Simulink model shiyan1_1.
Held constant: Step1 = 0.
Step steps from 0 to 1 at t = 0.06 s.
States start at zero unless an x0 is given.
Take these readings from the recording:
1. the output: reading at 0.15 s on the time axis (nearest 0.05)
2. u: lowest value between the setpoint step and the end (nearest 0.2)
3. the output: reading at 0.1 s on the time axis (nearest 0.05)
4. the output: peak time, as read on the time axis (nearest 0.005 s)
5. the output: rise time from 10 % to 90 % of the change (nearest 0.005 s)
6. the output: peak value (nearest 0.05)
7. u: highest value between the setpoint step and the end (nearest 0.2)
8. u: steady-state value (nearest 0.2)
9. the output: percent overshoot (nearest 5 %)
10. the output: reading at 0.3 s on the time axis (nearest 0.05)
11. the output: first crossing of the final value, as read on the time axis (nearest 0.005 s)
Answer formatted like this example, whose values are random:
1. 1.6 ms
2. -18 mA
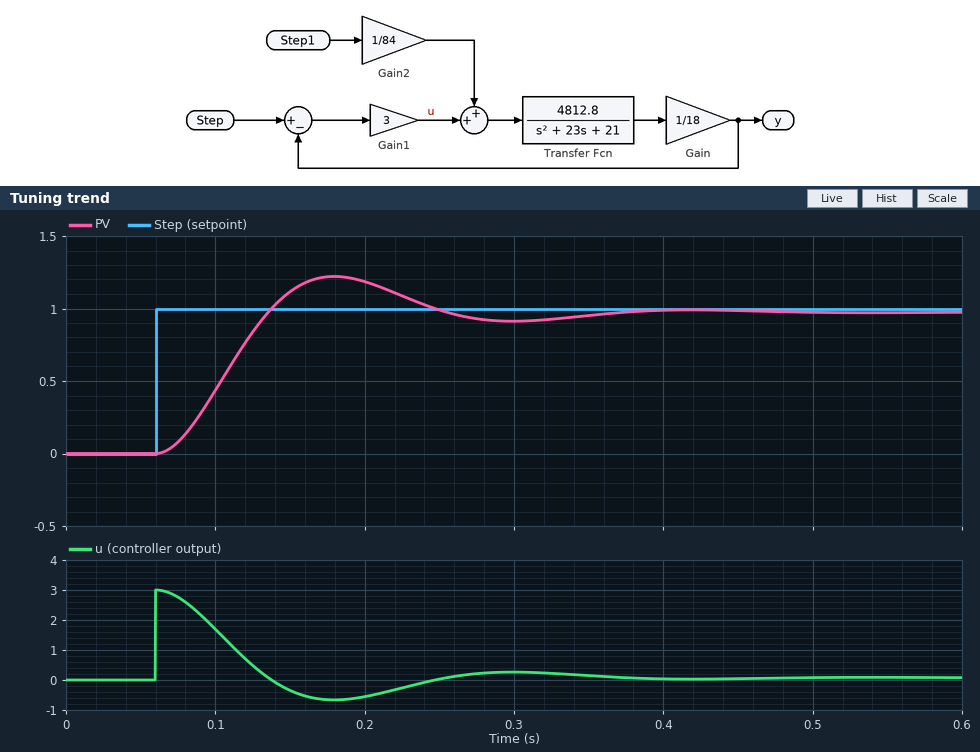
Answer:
1. 1.10
2. -0.6
3. 0.45
4. 0.180 s
5. 0.050 s
6. 1.20
7. 3.0
8. 0.0
9. 25 %
10. 0.90
11. 0.135 s
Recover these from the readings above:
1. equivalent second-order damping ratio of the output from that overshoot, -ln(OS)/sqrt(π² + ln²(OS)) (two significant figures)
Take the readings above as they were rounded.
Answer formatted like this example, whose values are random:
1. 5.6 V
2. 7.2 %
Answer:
1. 0.40
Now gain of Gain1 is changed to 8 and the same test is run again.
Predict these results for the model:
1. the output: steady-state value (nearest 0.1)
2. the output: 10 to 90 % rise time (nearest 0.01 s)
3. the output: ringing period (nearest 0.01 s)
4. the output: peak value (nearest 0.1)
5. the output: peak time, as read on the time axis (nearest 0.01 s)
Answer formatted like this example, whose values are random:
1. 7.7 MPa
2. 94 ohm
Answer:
1. 1.0
2. 0.03 s
3. 0.14 s
4. 1.4
5. 0.13 s
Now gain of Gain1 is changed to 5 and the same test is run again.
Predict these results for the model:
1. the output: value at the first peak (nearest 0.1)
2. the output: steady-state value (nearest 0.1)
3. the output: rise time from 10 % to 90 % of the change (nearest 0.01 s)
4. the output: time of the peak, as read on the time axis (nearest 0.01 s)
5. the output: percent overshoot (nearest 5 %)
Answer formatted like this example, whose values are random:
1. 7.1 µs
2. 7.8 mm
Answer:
1. 1.3
2. 1.0
3. 0.04 s
4. 0.15 s
5. 35 %
